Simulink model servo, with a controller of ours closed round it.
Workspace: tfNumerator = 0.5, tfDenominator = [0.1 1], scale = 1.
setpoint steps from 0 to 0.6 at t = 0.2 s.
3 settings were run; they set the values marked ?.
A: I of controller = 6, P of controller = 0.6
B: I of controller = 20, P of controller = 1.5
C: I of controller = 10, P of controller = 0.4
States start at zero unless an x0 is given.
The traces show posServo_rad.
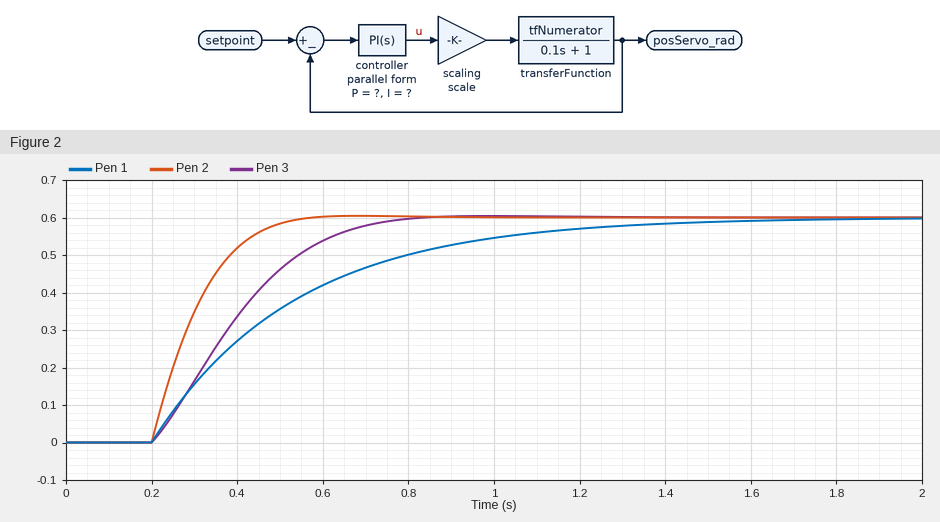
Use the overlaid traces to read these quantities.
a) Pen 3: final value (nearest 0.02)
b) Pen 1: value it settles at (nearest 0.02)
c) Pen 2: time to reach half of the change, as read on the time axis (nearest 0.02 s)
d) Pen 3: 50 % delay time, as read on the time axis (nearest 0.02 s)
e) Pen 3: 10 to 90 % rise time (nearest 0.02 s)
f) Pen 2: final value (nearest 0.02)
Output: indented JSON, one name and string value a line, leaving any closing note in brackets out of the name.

{
  "Pen 3: final value": "0.60",
  "Pen 1: value it settles at": "0.60",
  "Pen 2: time to reach half of the change, as read on the time axis": "0.28 s",
  "Pen 3: 50 % delay time, as read on the time axis": "0.38 s",
  "Pen 3: 10 to 90 % rise time": "0.36 s",
  "Pen 2: final value": "0.60"
}
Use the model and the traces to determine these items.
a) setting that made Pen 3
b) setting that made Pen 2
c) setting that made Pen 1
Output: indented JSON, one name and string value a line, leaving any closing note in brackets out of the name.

{
  "setting that made Pen 3": "C",
  "setting that made Pen 2": "B",
  "setting that made Pen 1": "A"
}
